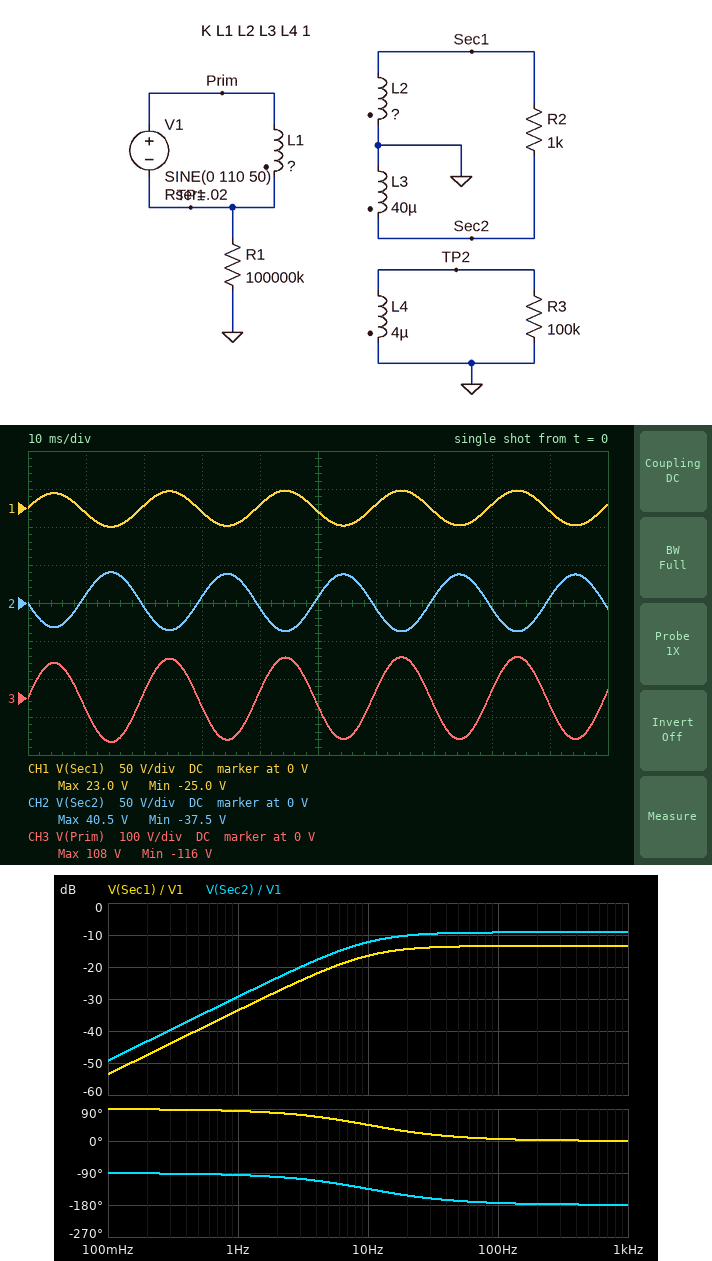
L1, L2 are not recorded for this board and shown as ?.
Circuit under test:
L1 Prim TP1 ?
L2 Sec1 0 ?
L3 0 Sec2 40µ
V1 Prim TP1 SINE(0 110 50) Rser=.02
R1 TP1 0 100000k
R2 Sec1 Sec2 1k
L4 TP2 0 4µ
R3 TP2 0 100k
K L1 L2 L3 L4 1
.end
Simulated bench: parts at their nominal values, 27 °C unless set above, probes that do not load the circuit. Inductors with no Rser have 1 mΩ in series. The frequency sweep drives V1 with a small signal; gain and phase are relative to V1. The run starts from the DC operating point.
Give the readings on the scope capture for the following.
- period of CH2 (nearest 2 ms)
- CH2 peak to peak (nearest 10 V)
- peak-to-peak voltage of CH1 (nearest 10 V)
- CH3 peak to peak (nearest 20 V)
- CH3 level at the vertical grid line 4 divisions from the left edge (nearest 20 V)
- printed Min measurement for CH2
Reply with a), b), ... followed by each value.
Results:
a) 20 ms
b) 80 V
c) 50 V
d) 220 V
e) 20 V
f) -37.5 V
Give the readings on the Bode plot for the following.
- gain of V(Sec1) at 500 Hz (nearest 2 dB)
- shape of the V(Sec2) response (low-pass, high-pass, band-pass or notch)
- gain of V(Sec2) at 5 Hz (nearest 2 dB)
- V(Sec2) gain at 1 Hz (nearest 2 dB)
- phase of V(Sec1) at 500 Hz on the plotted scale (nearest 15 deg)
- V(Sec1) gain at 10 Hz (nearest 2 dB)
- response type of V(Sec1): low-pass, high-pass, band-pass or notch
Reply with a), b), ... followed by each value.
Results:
a) -14 dB
b) high-pass
c) -16 dB
d) -30 dB
e) 0 deg
f) -16 dB
g) high-pass
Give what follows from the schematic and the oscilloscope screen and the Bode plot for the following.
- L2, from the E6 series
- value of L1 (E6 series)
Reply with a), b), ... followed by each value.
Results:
a) 15 µH
b) 330 µH
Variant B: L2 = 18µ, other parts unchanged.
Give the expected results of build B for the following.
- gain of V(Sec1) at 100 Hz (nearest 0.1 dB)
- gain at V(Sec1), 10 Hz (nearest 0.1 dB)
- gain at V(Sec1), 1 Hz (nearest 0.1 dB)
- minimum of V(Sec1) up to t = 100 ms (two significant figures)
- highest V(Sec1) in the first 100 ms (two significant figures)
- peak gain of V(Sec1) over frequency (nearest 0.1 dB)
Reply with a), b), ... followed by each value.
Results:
a) -12.7 dB
b) -15.7 dB
c) -32.8 dB
d) -27 V
e) 25 V
f) -12.6 dB
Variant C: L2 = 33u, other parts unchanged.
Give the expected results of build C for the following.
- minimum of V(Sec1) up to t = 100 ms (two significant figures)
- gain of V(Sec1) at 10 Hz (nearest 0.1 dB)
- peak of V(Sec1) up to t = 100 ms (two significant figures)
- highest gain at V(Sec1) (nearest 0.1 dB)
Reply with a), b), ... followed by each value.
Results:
a) -37 V
b) -13.1 dB
c) 34 V
d) -10.0 dB
